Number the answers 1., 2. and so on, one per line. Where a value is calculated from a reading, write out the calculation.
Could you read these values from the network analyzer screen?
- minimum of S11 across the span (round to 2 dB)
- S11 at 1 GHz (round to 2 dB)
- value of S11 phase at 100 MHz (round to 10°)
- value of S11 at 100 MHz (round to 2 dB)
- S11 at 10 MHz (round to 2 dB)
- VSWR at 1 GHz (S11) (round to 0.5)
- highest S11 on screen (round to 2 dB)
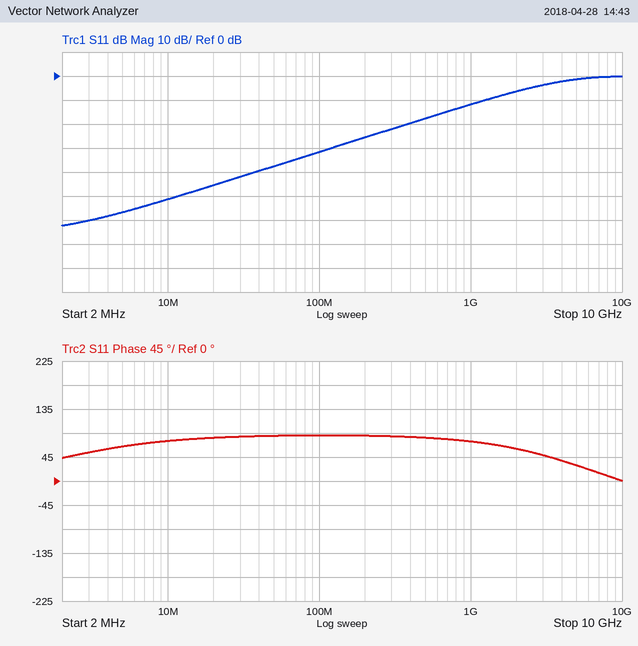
1. -62 dB
2. -12 dB
3. 90°
4. -32 dB
5. -52 dB
6. |Γ| = 10^(-12/20) = 0.2512; VSWR = (1 + 0.2512)/(1 − 0.2512) ≈ 1.67, so 1.5 to the nearest 0.5
7. 0 dB
